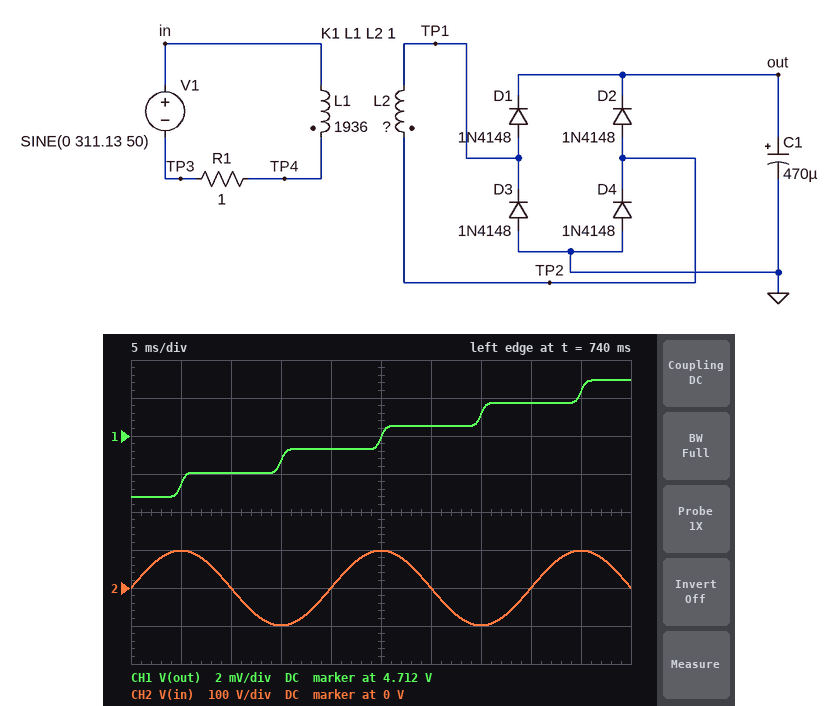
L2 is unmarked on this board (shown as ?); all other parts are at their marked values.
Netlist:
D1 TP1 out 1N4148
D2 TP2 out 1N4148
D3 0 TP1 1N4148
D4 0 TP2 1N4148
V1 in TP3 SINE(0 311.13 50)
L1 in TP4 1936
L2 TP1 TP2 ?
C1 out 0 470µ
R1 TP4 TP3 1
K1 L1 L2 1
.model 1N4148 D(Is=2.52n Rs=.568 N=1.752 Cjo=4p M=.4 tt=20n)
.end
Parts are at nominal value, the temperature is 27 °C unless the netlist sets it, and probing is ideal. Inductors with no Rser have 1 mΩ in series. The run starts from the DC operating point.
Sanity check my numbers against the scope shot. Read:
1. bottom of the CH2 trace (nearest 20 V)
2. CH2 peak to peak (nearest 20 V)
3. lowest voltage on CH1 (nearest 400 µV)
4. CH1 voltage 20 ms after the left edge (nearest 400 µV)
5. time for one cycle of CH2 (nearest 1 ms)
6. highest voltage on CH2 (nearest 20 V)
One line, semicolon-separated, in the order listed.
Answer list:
-100 V; 200 V; 4.7088 V; 4.7112 V; 20 ms; 100 V
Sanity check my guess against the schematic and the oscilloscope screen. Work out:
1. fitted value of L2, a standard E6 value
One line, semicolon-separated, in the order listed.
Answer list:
680 mH
